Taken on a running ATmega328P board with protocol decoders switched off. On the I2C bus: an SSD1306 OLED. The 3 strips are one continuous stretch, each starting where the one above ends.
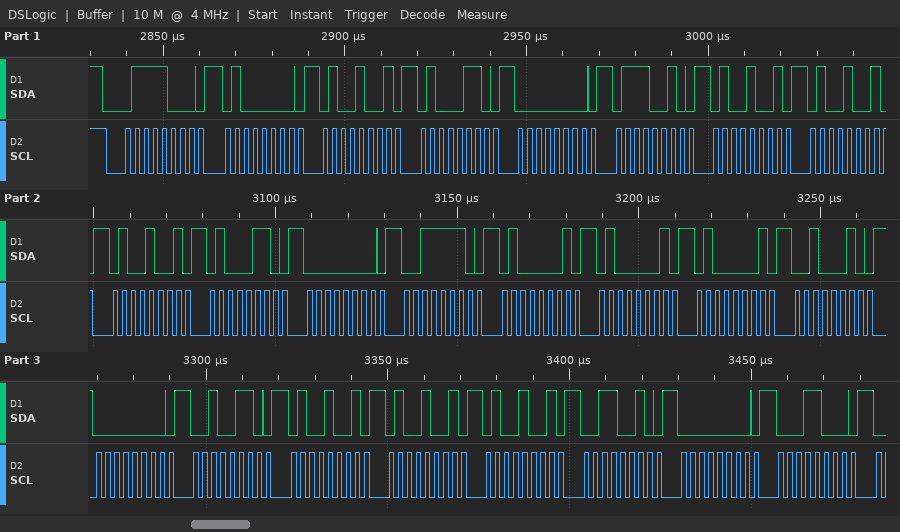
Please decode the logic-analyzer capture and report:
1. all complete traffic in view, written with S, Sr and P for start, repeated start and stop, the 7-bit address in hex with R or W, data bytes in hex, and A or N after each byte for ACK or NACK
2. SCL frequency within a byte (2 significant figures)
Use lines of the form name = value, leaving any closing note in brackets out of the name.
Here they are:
all complete traffic in view, written with S, Sr and P for start, repeated start and stop, the 7-bit address in hex with R or W, data bytes in hex, and A or N after each byte for ACK or NACK = S 3CW A 40 A 49 A 46 A 00 A 72 A 49 A 49 A 49 A 46 A 00 A 3E A 41 A 41 A 41 A 22 A 00 A 26 A 49 A 49 A 49 A 32 A 00 A 18 A
SCL frequency within a byte = 400 kHz
